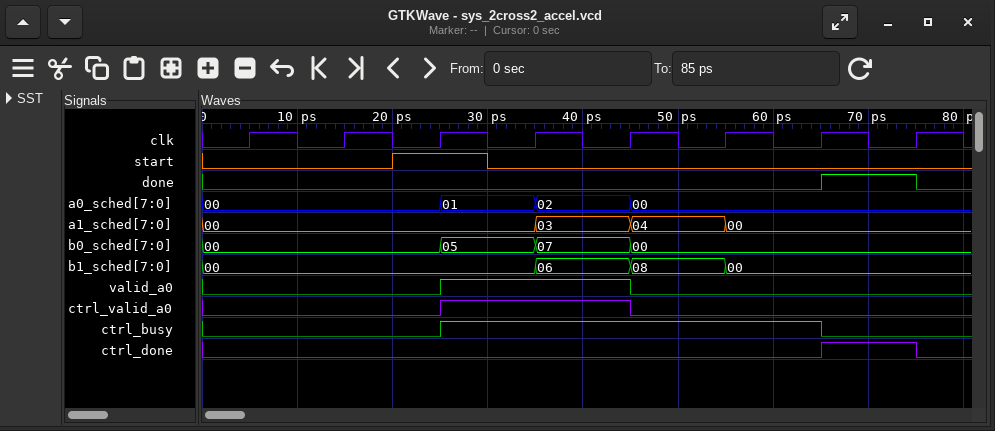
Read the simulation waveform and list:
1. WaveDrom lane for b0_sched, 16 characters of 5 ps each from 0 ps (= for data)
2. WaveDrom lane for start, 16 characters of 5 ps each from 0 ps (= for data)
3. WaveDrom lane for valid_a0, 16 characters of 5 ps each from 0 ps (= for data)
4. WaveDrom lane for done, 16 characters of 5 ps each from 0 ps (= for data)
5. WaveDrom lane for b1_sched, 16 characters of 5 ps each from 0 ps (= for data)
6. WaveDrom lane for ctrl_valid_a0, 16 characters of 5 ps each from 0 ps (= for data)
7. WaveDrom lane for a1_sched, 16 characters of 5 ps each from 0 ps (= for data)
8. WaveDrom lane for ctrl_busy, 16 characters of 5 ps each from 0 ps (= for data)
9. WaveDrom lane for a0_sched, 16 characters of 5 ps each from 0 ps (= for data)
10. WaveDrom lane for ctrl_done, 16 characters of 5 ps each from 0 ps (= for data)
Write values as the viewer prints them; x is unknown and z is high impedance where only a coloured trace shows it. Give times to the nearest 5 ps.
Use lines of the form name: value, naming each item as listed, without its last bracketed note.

WaveDrom lane for b0_sched, 16 characters of 5 ps each from 0 ps: {name: 'b0_sched', wave: '=....=.=.=......', data: '00 05 07 00'}
WaveDrom lane for start, 16 characters of 5 ps each from 0 ps: {name: 'start', wave: '0...1.0.........'}
WaveDrom lane for valid_a0, 16 characters of 5 ps each from 0 ps: {name: 'valid_a0', wave: '0....1...0......'}
WaveDrom lane for done, 16 characters of 5 ps each from 0 ps: {name: 'done', wave: '0............1.0'}
WaveDrom lane for b1_sched, 16 characters of 5 ps each from 0 ps: {name: 'b1_sched', wave: '=......=.=.=....', data: '00 06 08 00'}
WaveDrom lane for ctrl_valid_a0, 16 characters of 5 ps each from 0 ps: {name: 'ctrl_valid_a0', wave: '0....1...0......'}
WaveDrom lane for a1_sched, 16 characters of 5 ps each from 0 ps: {name: 'a1_sched', wave: '=......=.=.=....', data: '00 03 04 00'}
WaveDrom lane for ctrl_busy, 16 characters of 5 ps each from 0 ps: {name: 'ctrl_busy', wave: '0....1.......0..'}
WaveDrom lane for a0_sched, 16 characters of 5 ps each from 0 ps: {name: 'a0_sched', wave: '=....=.=.=......', data: '00 01 02 00'}
WaveDrom lane for ctrl_done, 16 characters of 5 ps each from 0 ps: {name: 'ctrl_done', wave: '0............1.0'}
